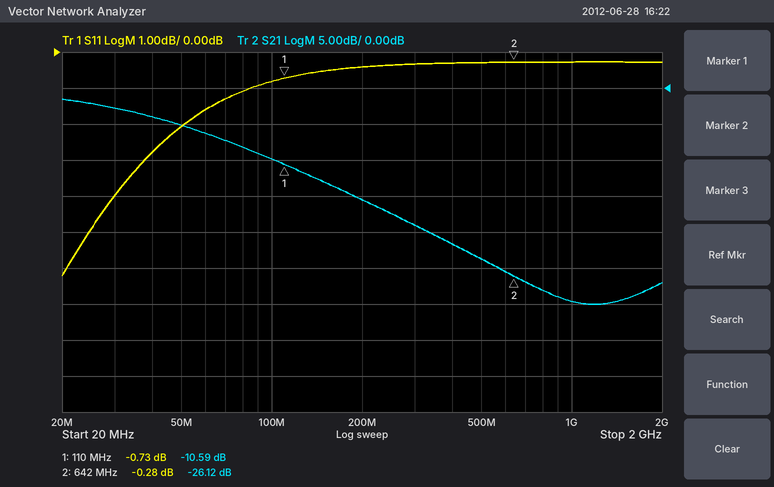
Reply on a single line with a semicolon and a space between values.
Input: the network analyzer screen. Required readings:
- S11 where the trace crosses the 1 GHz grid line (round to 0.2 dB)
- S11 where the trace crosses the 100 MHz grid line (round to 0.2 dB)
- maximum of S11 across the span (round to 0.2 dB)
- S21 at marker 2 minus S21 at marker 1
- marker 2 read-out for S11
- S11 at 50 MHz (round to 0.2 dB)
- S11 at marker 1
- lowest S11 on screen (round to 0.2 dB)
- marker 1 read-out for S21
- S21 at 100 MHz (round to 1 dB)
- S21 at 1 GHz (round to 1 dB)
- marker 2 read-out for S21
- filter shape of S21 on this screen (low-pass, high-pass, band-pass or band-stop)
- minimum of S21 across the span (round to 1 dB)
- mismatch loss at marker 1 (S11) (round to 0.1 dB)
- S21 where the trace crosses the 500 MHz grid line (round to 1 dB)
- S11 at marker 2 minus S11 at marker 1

-0.2 dB; -0.8 dB; -0.2 dB; -15.53 dB; -0.28 dB; -2.0 dB; -0.73 dB; -6.2 dB; -10.59 dB; -10 dB; -30 dB; -26.12 dB; low-pass; -30 dB; 8.1 dB; -24 dB; 0.45 dB
